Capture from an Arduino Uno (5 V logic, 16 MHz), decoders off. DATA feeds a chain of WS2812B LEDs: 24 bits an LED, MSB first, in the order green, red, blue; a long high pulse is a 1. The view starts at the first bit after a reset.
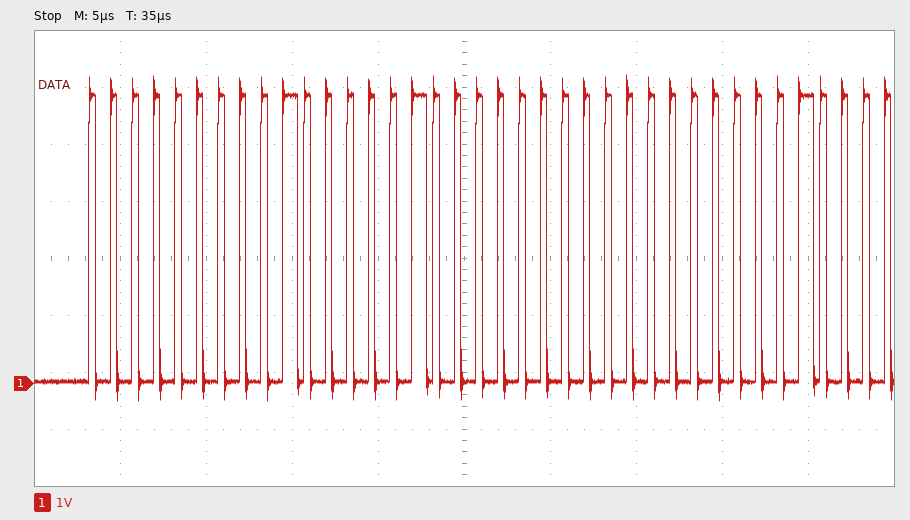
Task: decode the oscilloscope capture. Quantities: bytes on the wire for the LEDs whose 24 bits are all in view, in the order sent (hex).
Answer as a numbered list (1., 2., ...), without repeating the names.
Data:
1. 00 41 00
